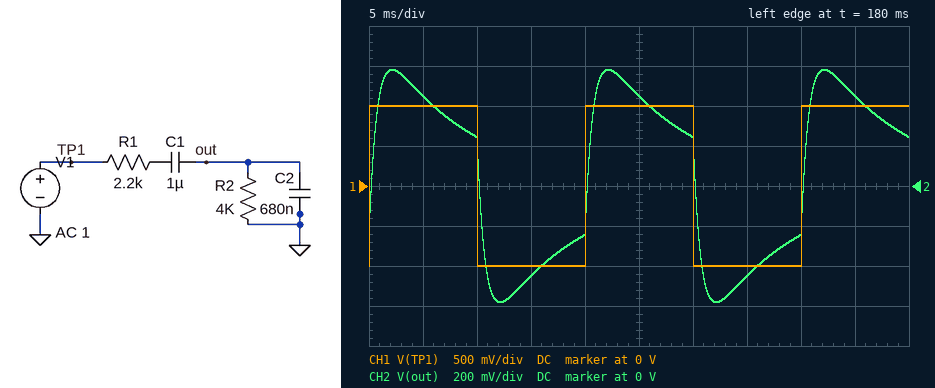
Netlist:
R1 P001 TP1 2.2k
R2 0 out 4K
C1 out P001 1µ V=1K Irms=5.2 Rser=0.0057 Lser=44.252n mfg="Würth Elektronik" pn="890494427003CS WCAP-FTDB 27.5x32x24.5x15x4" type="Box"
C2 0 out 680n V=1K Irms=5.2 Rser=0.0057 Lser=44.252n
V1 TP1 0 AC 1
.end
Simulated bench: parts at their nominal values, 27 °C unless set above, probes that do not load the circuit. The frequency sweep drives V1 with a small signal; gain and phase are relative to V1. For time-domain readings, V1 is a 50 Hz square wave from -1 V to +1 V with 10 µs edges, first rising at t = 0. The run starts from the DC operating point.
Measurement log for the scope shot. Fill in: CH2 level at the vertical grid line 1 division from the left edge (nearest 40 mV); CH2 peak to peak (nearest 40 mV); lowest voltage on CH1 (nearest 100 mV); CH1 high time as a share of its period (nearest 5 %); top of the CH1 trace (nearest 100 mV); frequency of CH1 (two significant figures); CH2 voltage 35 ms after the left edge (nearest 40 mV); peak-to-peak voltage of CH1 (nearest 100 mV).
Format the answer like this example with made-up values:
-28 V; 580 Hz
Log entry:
440 mV; 1.16 V; -1.0 V; 50 %; 1.0 V; 50 Hz; -440 mV; 2.0 V
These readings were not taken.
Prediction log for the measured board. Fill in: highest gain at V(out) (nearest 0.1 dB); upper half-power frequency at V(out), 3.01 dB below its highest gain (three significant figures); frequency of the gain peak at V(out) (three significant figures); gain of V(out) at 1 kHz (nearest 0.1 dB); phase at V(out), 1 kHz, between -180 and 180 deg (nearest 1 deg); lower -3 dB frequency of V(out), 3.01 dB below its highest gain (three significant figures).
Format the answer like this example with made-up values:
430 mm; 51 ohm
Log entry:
-7.0 dB; 254 Hz; 65.1 Hz; -19.7 dB; -77 deg; 16.7 Hz
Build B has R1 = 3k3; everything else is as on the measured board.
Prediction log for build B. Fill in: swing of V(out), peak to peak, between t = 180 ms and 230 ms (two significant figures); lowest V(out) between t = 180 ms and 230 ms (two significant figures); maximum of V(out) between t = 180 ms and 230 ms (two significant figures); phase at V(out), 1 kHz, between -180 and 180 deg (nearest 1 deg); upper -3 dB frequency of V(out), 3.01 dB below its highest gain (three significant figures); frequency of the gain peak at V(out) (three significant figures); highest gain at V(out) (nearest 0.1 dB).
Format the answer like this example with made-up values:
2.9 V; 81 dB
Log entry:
980 mV; -490 mV; 490 mV; -80 deg; 192 Hz; 53.1 Hz; -8.0 dB
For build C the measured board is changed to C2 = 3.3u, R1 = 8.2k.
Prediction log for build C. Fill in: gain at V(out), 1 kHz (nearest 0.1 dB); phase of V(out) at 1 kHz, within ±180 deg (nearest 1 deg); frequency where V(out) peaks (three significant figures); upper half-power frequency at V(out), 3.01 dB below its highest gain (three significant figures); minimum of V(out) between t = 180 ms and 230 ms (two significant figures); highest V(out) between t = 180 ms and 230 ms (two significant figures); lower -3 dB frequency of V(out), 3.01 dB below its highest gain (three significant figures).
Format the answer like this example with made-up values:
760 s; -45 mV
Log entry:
-44.6 dB; -88 deg; 15.3 Hz; 42.8 Hz; -130 mV; 130 mV; 5.47 Hz
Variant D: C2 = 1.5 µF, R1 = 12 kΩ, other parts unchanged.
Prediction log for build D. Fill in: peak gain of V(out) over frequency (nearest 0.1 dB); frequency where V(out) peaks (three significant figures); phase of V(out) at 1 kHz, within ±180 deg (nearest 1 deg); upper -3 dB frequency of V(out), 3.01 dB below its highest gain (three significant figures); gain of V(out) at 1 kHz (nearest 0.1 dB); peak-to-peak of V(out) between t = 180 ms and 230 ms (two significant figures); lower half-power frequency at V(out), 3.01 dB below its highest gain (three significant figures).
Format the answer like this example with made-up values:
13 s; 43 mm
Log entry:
-14.8 dB; 18.8 Hz; -87 deg; 55.0 Hz; -41.1 dB; 330 mV; 6.39 Hz
